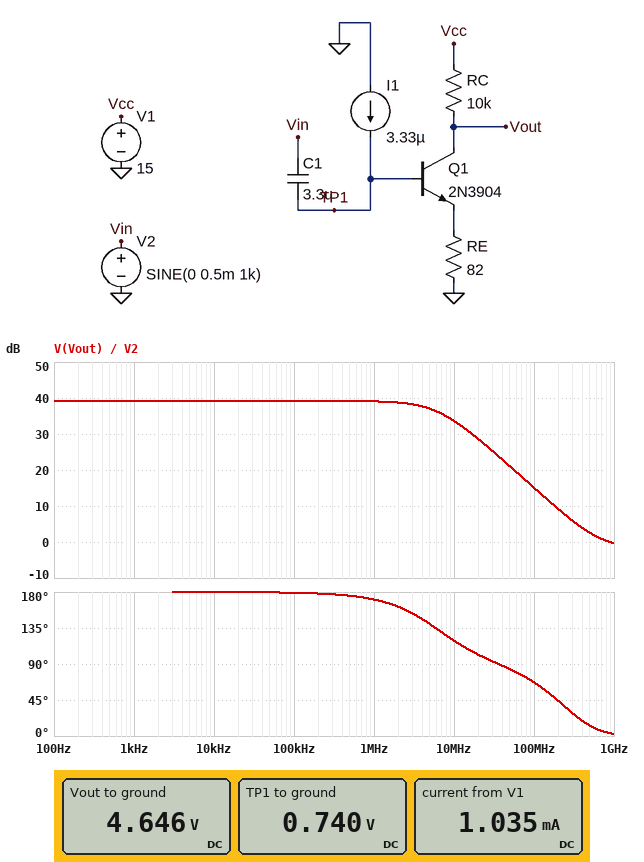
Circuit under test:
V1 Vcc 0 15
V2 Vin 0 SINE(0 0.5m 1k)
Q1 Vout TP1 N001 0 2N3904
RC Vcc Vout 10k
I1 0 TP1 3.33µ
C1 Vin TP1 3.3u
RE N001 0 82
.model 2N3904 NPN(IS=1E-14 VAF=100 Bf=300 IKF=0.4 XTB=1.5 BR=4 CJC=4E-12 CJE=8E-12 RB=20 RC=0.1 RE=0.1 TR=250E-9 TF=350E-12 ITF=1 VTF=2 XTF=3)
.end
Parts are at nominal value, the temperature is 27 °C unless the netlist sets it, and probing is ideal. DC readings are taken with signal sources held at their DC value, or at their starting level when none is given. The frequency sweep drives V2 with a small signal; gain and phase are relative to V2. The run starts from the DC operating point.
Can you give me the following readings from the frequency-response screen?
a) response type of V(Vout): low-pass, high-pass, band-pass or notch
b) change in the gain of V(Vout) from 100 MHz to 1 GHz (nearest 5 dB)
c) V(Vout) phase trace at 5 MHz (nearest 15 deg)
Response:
low-pass
-15 dB
135 deg
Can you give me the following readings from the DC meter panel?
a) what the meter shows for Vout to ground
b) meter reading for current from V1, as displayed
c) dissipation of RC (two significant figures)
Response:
4.646 V
1.035 mA
11 mW
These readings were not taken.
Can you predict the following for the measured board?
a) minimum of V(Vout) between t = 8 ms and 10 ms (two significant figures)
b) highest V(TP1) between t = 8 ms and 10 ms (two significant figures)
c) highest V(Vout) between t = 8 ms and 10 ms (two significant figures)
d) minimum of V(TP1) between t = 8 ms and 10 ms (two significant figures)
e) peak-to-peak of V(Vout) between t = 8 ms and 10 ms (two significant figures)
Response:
4.6 V
740 mV
4.7 V
740 mV
91 mV
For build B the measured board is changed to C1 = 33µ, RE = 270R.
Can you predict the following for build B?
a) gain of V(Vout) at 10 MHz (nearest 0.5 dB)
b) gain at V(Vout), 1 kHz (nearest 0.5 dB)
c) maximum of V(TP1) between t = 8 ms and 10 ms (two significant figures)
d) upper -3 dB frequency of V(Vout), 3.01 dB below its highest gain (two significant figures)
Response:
25.5 dB
30.5 dB
940 mV
6.8 MHz
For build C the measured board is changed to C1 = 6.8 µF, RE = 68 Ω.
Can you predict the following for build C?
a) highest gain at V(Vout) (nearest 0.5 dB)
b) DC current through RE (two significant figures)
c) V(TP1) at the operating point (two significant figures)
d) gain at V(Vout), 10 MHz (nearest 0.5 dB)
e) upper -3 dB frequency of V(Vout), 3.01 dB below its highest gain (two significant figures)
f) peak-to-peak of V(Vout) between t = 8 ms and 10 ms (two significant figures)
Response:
40.5 dB
1.0 mA
730 mV
34.5 dB
6.1 MHz
100 mV
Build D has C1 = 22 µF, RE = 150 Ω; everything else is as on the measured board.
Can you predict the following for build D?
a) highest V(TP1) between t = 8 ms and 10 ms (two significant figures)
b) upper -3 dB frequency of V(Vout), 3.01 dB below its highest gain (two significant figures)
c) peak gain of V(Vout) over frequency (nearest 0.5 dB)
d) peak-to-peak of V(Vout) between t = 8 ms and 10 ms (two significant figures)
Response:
810 mV
6.6 MHz
35.0 dB
56 mV
